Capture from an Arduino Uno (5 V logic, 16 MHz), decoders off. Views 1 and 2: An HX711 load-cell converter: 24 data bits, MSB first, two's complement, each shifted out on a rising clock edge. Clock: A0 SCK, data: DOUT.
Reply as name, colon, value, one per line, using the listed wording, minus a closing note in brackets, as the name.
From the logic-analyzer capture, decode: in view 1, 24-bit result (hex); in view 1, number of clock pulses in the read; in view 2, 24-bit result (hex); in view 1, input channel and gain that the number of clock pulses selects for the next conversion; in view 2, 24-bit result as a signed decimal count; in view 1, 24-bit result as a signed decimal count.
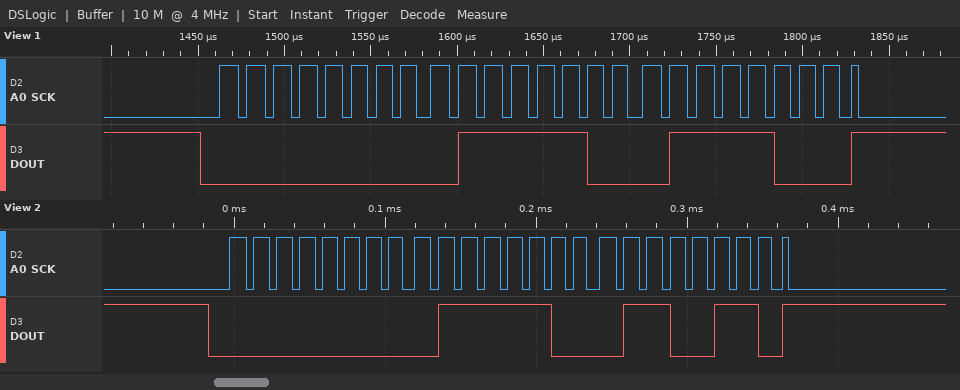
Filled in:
in view 1, 24-bit result: 0x007C78
in view 1, number of clock pulses in the read: 25
in view 2, 24-bit result: 0x007C66
in view 1, input channel and gain that the number of clock pulses selects for the next conversion: channel A, gain 128
in view 2, 24-bit result as a signed decimal count: 31846
in view 1, 24-bit result as a signed decimal count: 31864
